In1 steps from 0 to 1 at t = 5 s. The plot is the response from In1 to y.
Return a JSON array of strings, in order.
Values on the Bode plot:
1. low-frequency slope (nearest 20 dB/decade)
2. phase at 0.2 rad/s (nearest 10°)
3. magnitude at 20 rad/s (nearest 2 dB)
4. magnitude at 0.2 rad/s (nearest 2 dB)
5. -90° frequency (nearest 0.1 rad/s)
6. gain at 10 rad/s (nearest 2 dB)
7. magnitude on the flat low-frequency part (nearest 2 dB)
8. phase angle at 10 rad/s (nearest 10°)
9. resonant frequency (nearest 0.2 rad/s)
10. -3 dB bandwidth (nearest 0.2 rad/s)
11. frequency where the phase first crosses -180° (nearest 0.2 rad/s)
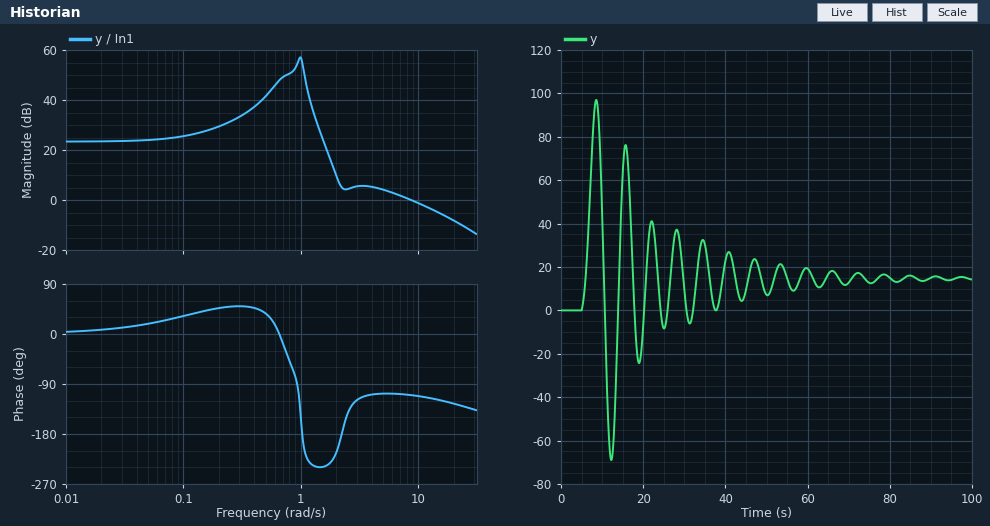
["0 dB/decade", "50°", "-8 dB", "30 dB", "0.9 rad/s", "-2 dB", "24 dB", "-110°", "1.0 rad/s", "1.6 rad/s", "1.0 rad/s"]
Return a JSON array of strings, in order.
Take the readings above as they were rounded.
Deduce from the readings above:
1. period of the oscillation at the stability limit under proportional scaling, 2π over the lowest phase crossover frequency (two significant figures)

["6.3 s"]
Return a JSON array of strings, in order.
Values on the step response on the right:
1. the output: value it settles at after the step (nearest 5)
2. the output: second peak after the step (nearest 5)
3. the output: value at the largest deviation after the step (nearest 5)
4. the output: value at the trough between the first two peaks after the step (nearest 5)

["15", "75", "95", "-70"]
